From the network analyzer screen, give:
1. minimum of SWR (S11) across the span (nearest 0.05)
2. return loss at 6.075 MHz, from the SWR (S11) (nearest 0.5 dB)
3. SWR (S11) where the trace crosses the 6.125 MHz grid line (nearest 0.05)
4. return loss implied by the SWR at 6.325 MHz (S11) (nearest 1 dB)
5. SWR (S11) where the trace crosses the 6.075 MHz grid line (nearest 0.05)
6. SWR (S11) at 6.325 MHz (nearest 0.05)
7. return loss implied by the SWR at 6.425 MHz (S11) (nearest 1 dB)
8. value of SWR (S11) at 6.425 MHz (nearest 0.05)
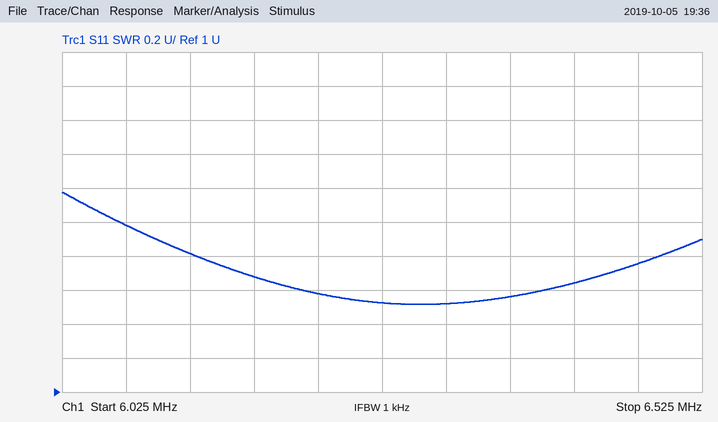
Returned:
1.50
9.5 dB
1.80
14 dB
2.00
1.50
12 dB
1.65
